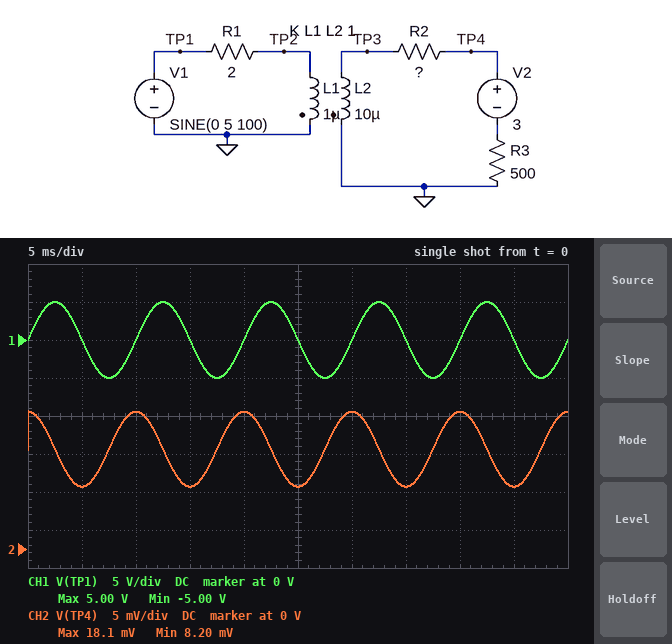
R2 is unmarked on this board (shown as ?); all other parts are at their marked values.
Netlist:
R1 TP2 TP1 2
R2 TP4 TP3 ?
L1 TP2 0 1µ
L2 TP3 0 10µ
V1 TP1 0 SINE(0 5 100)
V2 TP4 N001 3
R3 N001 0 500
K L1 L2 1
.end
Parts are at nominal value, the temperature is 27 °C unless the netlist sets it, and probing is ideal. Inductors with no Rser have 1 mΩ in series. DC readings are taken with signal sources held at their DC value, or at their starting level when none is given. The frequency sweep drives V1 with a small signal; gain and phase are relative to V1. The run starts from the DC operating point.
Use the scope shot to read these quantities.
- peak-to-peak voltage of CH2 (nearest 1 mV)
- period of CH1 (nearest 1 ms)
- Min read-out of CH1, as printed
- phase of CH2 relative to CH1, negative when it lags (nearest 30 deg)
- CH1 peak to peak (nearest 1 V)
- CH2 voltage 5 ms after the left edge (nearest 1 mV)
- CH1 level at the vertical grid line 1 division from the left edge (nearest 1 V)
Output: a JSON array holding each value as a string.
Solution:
["10 mV", "10 ms", "-5.00 V", "90 deg", "10 V", "8 mV", "0 V"]
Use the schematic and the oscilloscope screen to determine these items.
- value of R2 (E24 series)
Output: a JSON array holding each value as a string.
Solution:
["2.2 Ω"]
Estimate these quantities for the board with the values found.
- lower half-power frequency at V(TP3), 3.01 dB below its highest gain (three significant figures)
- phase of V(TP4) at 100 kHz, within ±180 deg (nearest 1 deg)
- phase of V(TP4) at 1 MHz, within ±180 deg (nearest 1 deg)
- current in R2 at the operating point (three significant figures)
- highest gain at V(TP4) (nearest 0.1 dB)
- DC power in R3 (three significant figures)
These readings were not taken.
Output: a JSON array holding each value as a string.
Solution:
["306 kHz", "72 deg", "17 deg", "5.97 mA", "9.6 dB", "17.8 mW"]
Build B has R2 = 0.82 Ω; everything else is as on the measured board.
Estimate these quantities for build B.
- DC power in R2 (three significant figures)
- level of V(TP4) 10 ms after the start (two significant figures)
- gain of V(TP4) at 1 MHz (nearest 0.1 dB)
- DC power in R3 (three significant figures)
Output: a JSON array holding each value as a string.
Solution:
["29.4 µW", "9.9 mV", "9.3 dB", "17.9 mW"]
